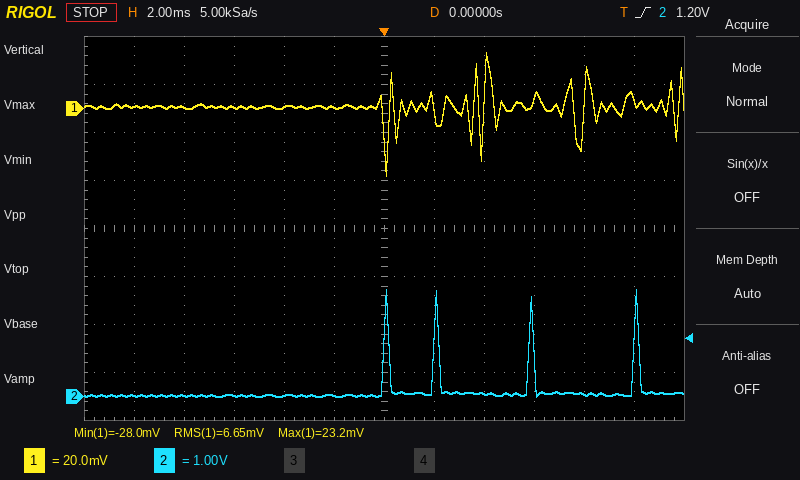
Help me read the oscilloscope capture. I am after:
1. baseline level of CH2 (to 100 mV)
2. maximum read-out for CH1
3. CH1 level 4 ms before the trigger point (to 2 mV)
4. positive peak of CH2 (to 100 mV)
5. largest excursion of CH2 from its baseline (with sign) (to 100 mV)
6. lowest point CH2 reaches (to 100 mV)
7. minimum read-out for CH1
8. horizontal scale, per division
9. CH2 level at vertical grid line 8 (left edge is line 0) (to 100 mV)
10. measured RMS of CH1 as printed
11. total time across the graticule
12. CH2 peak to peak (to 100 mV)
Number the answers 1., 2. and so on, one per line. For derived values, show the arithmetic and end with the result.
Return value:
1. 0.0 V
2. 23.2 mV
3. 0 mV
4. 2.2 V
5. 2.2 V − (0.0 V) = +2.2 V
6. 0.0 V
7. -28.0 mV
8. 2 ms
9. 100 mV
10. 6.65 mV
11. 24 ms
12. 2.2 V − (0.0 V) = 2.2 V
